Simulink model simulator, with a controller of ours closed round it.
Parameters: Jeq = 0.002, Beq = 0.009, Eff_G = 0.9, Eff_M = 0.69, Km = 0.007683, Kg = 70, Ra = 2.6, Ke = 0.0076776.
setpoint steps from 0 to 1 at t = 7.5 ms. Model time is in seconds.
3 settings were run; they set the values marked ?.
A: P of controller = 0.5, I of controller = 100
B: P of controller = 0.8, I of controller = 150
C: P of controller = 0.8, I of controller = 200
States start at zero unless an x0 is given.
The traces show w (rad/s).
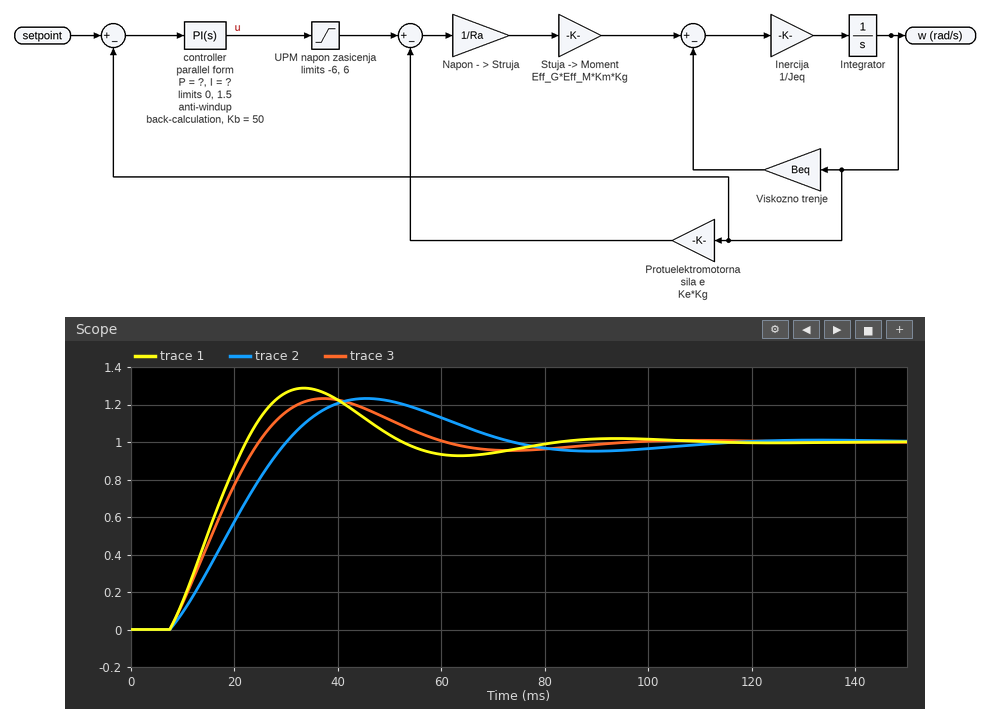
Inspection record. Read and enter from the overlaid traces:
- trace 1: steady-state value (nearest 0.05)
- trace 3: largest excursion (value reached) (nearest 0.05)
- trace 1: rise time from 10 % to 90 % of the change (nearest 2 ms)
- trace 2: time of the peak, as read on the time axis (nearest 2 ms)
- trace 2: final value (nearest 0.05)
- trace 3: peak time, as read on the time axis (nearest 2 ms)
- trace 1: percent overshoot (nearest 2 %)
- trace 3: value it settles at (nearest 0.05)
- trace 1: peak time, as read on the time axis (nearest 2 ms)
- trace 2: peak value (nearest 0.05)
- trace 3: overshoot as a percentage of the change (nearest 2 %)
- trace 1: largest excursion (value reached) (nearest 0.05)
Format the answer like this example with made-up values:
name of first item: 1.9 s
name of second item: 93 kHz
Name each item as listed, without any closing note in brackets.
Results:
trace 1: steady-state value: 1.00
trace 3: largest excursion (value reached): 1.25
trace 1: rise time from 10 % to 90 % of the change: 12 ms
trace 2: time of the peak, as read on the time axis: 46 ms
trace 2: final value: 1.00
trace 3: peak time, as read on the time axis: 38 ms
trace 1: percent overshoot: 28 %
trace 3: value it settles at: 1.00
trace 1: peak time, as read on the time axis: 34 ms
trace 2: peak value: 1.25
trace 3: overshoot as a percentage of the change: 24 %
trace 1: largest excursion (value reached): 1.30
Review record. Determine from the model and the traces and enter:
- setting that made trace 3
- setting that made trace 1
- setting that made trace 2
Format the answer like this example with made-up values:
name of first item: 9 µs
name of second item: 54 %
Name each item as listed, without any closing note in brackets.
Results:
setting that made trace 3: B
setting that made trace 1: C
setting that made trace 2: A
